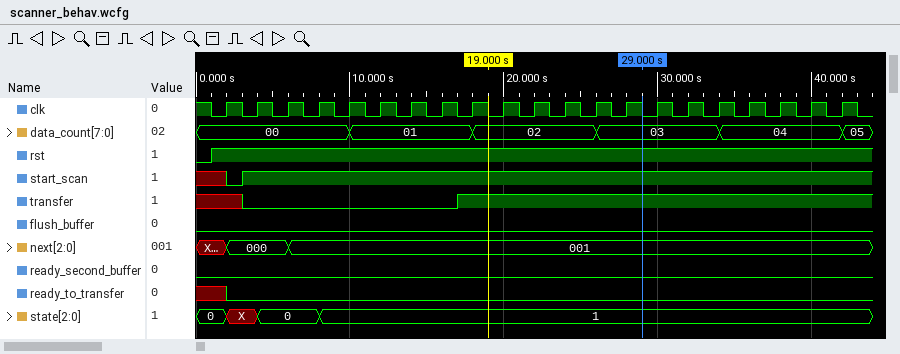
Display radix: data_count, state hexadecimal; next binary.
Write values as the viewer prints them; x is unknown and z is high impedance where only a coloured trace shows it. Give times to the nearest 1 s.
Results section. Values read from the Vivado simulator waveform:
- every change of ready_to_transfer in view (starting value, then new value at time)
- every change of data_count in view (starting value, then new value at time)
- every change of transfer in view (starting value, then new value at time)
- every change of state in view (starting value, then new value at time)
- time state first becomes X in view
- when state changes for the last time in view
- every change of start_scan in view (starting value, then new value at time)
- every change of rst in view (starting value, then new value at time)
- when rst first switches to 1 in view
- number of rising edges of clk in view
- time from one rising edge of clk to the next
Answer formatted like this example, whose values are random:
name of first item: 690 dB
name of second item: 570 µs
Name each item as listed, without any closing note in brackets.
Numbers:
every change of ready_to_transfer in view: x, 0 at 2 s
every change of data_count in view: 00, 01 at 10 s, 02 at 18 s, 03 at 26 s, 04 at 34 s, 05 at 42 s
every change of transfer in view: x, 0 at 3 s, 1 at 17 s
every change of state in view: 0, X at 2 s, 0 at 4 s, 1 at 8 s
time state first becomes X in view: 2 s
when state changes for the last time in view: 8 s
every change of start_scan in view: x, 0 at 2 s, 1 at 3 s
every change of rst in view: 0, 1 at 1 s
when rst first switches to 1 in view: 1 s
number of rising edges of clk in view: 21
time from one rising edge of clk to the next: 2 s
